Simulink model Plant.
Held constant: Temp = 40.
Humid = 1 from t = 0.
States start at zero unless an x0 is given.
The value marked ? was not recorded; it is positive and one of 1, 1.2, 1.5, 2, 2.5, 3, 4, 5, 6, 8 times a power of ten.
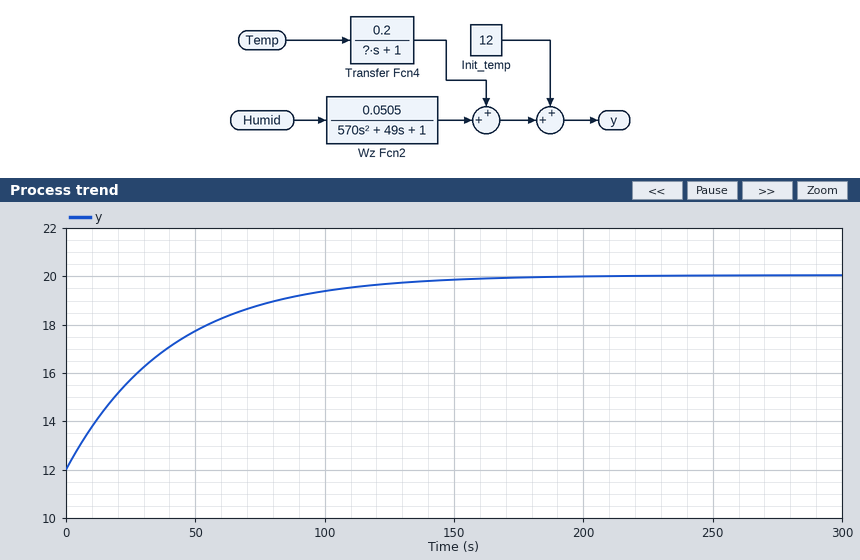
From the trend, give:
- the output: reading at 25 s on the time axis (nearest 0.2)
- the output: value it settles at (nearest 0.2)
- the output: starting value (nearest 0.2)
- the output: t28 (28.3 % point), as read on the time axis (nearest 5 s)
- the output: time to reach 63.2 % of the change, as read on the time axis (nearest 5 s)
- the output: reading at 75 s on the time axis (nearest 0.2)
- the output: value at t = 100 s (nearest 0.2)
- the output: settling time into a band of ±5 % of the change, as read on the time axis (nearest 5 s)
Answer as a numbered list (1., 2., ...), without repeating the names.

1. 15.8
2. 20.0
3. 12.0
4. 15 s
5. 40 s
6. 18.8
7. 19.4
8. 120 s
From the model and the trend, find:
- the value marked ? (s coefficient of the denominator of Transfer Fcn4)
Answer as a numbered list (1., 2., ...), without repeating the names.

1. 40
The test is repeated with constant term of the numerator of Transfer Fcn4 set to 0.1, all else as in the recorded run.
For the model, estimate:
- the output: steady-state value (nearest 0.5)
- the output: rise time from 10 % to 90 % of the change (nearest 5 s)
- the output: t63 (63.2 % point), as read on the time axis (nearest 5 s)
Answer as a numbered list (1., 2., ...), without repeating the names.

1. 16.0
2. 90 s
3. 40 s
